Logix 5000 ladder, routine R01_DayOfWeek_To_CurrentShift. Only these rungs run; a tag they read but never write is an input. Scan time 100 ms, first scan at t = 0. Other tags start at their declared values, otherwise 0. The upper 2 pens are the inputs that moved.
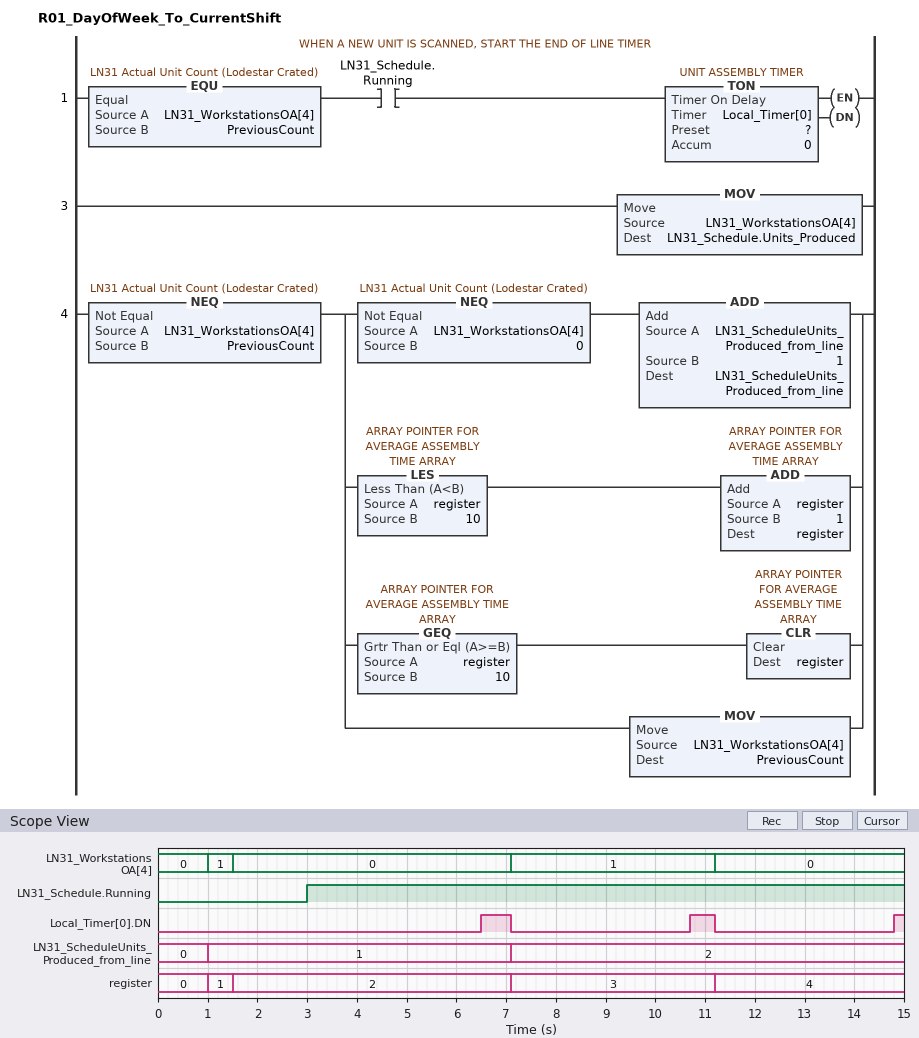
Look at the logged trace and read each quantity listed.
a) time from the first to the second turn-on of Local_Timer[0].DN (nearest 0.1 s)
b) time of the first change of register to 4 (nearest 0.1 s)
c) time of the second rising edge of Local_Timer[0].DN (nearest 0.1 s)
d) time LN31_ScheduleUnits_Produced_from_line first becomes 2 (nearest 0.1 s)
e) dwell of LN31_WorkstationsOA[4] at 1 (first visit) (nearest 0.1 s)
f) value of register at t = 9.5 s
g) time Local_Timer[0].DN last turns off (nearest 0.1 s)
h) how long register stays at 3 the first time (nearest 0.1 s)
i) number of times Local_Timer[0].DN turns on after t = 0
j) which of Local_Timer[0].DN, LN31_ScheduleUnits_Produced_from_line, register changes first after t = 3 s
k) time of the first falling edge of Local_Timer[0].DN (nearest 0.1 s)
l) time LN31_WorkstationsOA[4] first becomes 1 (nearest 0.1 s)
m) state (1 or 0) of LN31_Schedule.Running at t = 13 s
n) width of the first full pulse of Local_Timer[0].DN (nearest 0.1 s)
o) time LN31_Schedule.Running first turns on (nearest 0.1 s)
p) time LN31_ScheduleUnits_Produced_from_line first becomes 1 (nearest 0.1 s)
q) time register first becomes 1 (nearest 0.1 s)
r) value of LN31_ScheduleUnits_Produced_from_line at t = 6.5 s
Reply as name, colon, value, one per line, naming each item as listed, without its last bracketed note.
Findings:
time from the first to the second turn-on of Local_Timer[0].DN: 4.2 s
time of the first change of register to 4: 11.2 s
time of the second rising edge of Local_Timer[0].DN: 10.7 s
time LN31_ScheduleUnits_Produced_from_line first becomes 2: 7.1 s
dwell of LN31_WorkstationsOA[4] at 1 (first visit): 0.5 s
value of register at t = 9.5 s: 3
time Local_Timer[0].DN last turns off: 11.2 s
how long register stays at 3 the first time: 4.1 s
number of times Local_Timer[0].DN turns on after t = 0: 3
which of Local_Timer[0].DN, LN31_ScheduleUnits_Produced_from_line, register changes first after t = 3 s: Local_Timer[0].DN
time of the first falling edge of Local_Timer[0].DN: 7.1 s
time LN31_WorkstationsOA[4] first becomes 1: 1.0 s
state (1 or 0) of LN31_Schedule.Running at t = 13 s: 1
width of the first full pulse of Local_Timer[0].DN: 0.6 s
time LN31_Schedule.Running first turns on: 3.0 s
time LN31_ScheduleUnits_Produced_from_line first becomes 1: 1.0 s
time register first becomes 1: 1.0 s
value of LN31_ScheduleUnits_Produced_from_line at t = 6.5 s: 1
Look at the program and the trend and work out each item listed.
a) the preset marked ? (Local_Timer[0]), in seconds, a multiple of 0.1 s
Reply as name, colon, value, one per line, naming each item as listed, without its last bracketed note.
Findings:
the preset marked ? (Local_Timer[0]), in seconds, a multiple of 0.1 s: 3.5 s
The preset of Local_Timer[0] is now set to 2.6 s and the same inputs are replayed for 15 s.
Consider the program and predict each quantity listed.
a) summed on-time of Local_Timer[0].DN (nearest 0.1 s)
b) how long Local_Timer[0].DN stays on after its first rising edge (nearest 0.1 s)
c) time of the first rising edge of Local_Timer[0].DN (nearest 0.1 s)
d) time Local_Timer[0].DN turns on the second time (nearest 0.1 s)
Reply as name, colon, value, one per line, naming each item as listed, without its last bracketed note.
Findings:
summed on-time of Local_Timer[0].DN: 4.0 s
how long Local_Timer[0].DN stays on after its first rising edge: 1.5 s
time of the first rising edge of Local_Timer[0].DN: 5.6 s
time Local_Timer[0].DN turns on the second time: 9.8 s
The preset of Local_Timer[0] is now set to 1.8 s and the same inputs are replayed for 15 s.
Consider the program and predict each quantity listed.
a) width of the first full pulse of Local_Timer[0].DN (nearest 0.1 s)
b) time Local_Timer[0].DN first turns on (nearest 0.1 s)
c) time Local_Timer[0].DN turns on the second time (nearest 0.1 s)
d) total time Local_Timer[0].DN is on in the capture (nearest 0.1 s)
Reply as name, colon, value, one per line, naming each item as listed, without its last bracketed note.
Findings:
width of the first full pulse of Local_Timer[0].DN: 2.3 s
time Local_Timer[0].DN first turns on: 4.8 s
time Local_Timer[0].DN turns on the second time: 9.0 s
total time Local_Timer[0].DN is on in the capture: 6.4 s
